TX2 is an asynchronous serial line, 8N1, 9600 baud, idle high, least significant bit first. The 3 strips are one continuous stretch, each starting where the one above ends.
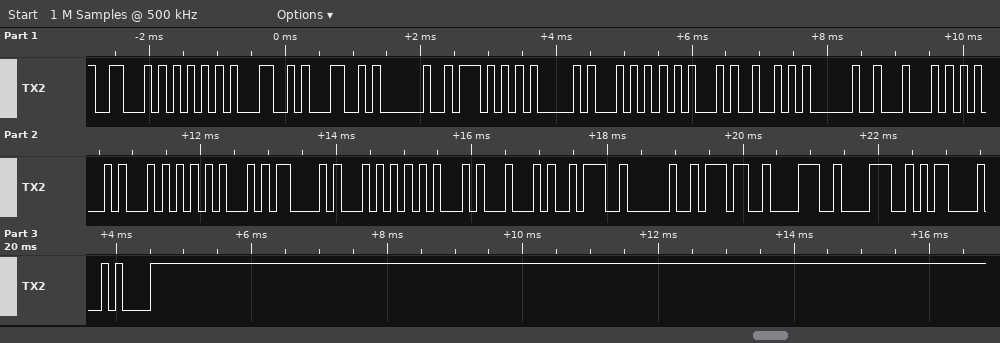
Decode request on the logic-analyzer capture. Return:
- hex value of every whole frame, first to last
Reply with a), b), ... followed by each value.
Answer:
a) 46 55 4C 4C 20 57 41 54 45 52 20 44 45 54 45 43 54 45 44 3A 20 37 38 38 0D 0A
